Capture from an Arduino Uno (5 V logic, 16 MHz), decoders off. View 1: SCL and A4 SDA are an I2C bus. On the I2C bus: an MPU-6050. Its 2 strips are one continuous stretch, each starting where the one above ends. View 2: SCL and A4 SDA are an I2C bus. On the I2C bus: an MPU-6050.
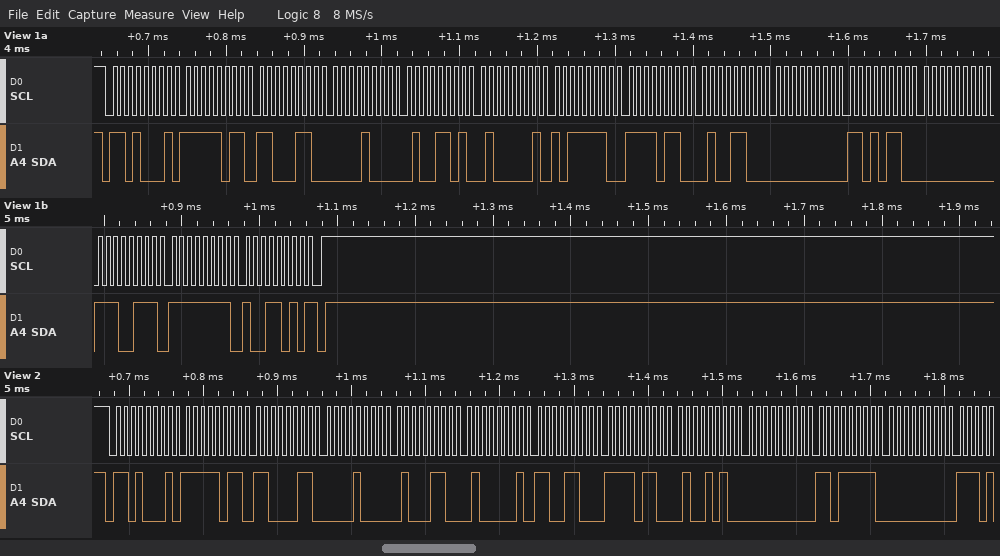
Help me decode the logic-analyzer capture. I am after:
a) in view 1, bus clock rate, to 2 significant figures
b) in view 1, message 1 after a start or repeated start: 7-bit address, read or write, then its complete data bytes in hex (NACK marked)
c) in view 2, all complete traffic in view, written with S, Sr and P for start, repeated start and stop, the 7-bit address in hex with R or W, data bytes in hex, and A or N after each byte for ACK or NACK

100 kHz
0x68 read: FB C6 08 4D 41 BE F6 4C 00 D6 00 E7 FF 9A NACK
S 68R A FB A C3 A 08 A 46 A 41 A CC A F6 A 4A A 00 A DF A 00 A
